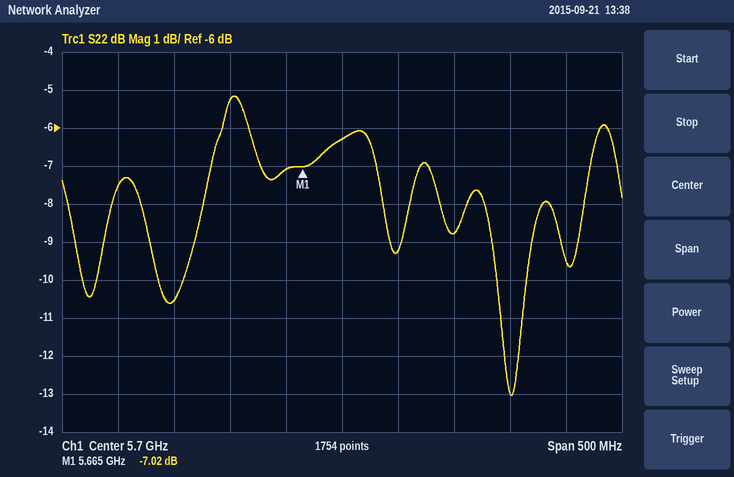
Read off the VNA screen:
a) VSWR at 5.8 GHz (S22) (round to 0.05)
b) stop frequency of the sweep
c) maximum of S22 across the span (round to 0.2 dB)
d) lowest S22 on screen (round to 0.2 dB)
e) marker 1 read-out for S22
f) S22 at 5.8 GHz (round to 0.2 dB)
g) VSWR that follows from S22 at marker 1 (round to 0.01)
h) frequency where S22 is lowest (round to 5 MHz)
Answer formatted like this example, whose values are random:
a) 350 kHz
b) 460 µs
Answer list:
a) 2.15
b) 5.95 GHz
c) -5.2 dB
d) -13.0 dB
e) -7.02 dB
f) -8.8 dB
g) 2.61
h) 5.850 GHz
